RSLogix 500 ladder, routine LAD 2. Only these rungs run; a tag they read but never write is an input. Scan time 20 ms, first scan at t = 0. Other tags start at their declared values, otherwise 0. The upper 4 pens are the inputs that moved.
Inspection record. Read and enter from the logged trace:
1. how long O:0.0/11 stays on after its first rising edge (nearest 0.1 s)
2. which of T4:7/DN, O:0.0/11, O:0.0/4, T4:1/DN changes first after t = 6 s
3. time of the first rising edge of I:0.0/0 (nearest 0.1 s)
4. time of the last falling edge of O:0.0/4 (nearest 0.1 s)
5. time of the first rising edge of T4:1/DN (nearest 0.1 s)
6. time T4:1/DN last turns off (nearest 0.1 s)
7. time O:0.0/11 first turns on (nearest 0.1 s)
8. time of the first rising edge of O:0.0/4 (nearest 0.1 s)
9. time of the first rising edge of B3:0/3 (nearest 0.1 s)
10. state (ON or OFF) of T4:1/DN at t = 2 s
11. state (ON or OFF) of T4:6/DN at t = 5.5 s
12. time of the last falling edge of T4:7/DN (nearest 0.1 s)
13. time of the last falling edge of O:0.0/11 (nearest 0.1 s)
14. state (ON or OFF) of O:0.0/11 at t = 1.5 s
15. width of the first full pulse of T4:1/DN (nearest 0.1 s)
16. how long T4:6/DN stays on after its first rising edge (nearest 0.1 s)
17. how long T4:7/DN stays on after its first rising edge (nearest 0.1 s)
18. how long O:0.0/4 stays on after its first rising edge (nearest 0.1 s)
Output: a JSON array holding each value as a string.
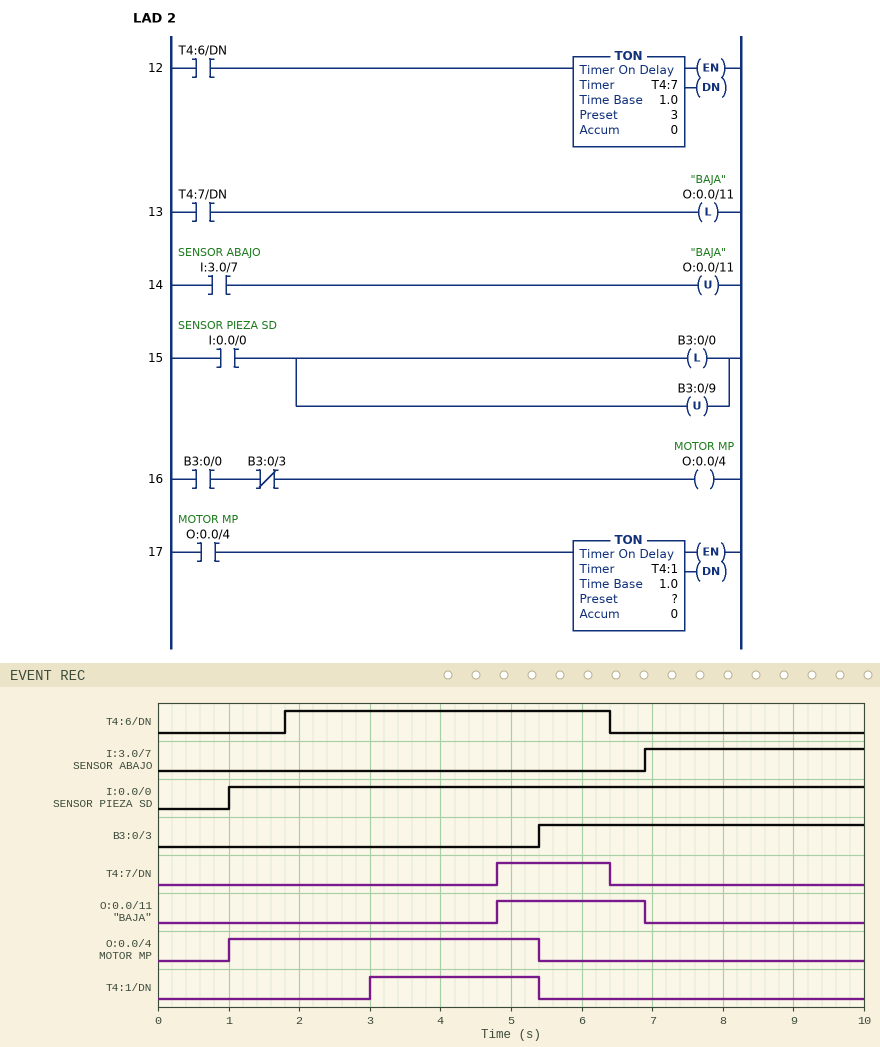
["2.1 s", "T4:7/DN", "1.0 s", "5.4 s", "3.0 s", "5.4 s", "4.8 s", "1.0 s", "5.4 s", "OFF", "ON", "6.4 s", "6.9 s", "OFF", "2.4 s", "4.6 s", "1.6 s", "4.4 s"]
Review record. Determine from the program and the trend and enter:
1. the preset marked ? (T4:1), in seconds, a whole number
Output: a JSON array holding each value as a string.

["2 s"]
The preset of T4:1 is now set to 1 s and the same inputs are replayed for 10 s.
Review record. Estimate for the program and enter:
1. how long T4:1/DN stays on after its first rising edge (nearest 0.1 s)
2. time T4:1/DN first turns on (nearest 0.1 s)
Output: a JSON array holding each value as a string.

["3.4 s", "2.0 s"]
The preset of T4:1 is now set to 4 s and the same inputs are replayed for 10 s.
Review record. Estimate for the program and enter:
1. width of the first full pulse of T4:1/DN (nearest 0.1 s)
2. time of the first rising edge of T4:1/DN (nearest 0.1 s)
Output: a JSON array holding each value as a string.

["0.4 s", "5.0 s"]
